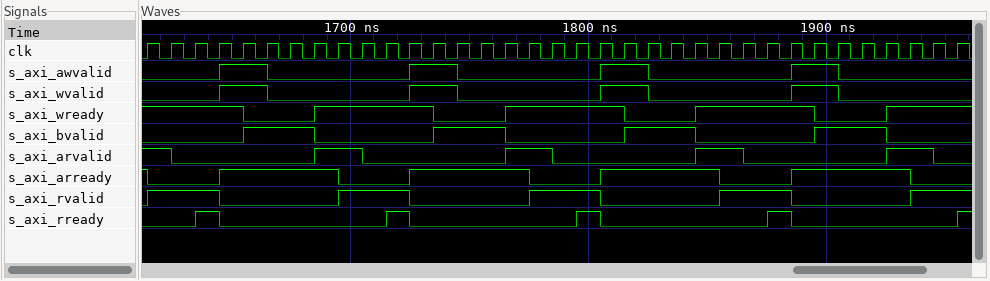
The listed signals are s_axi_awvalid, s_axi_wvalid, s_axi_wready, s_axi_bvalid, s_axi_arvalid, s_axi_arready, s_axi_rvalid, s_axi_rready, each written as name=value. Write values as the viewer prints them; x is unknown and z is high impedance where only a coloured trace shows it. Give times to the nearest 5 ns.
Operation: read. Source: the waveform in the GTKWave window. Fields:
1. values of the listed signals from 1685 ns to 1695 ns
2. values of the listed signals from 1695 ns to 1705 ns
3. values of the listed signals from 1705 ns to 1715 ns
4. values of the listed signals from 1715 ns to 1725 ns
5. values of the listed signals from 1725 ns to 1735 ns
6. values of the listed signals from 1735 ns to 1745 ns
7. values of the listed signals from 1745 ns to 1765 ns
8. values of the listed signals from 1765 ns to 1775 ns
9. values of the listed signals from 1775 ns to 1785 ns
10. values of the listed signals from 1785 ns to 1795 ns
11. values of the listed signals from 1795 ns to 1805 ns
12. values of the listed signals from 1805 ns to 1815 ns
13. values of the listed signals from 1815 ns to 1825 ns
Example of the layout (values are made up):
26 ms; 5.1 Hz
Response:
s_axi_awvalid=0, s_axi_wvalid=0, s_axi_wready=1, s_axi_bvalid=0, s_axi_arvalid=1, s_axi_arready=1, s_axi_rvalid=0, s_axi_rready=0; s_axi_awvalid=0, s_axi_wvalid=0, s_axi_wready=1, s_axi_bvalid=0, s_axi_arvalid=1, s_axi_arready=0, s_axi_rvalid=1, s_axi_rready=0; s_axi_awvalid=0, s_axi_wvalid=0, s_axi_wready=1, s_axi_bvalid=0, s_axi_arvalid=0, s_axi_arready=0, s_axi_rvalid=1, s_axi_rready=0; s_axi_awvalid=0, s_axi_wvalid=0, s_axi_wready=1, s_axi_bvalid=0, s_axi_arvalid=0, s_axi_arready=0, s_axi_rvalid=1, s_axi_rready=1; s_axi_awvalid=1, s_axi_wvalid=1, s_axi_wready=1, s_axi_bvalid=0, s_axi_arvalid=0, s_axi_arready=1, s_axi_rvalid=0, s_axi_rready=0; s_axi_awvalid=1, s_axi_wvalid=1, s_axi_wready=0, s_axi_bvalid=1, s_axi_arvalid=0, s_axi_arready=1, s_axi_rvalid=0, s_axi_rready=0; s_axi_awvalid=0, s_axi_wvalid=0, s_axi_wready=0, s_axi_bvalid=1, s_axi_arvalid=0, s_axi_arready=1, s_axi_rvalid=0, s_axi_rready=0; s_axi_awvalid=0, s_axi_wvalid=0, s_axi_wready=1, s_axi_bvalid=0, s_axi_arvalid=1, s_axi_arready=1, s_axi_rvalid=0, s_axi_rready=0; s_axi_awvalid=0, s_axi_wvalid=0, s_axi_wready=1, s_axi_bvalid=0, s_axi_arvalid=1, s_axi_arready=0, s_axi_rvalid=1, s_axi_rready=0; s_axi_awvalid=0, s_axi_wvalid=0, s_axi_wready=1, s_axi_bvalid=0, s_axi_arvalid=0, s_axi_arready=0, s_axi_rvalid=1, s_axi_rready=0; s_axi_awvalid=0, s_axi_wvalid=0, s_axi_wready=1, s_axi_bvalid=0, s_axi_arvalid=0, s_axi_arready=0, s_axi_rvalid=1, s_axi_rready=1; s_axi_awvalid=1, s_axi_wvalid=1, s_axi_wready=1, s_axi_bvalid=0, s_axi_arvalid=0, s_axi_arready=1, s_axi_rvalid=0, s_axi_rready=0; s_axi_awvalid=1, s_axi_wvalid=1, s_axi_wready=0, s_axi_bvalid=1, s_axi_arvalid=0, s_axi_arready=1, s_axi_rvalid=0, s_axi_rready=0
